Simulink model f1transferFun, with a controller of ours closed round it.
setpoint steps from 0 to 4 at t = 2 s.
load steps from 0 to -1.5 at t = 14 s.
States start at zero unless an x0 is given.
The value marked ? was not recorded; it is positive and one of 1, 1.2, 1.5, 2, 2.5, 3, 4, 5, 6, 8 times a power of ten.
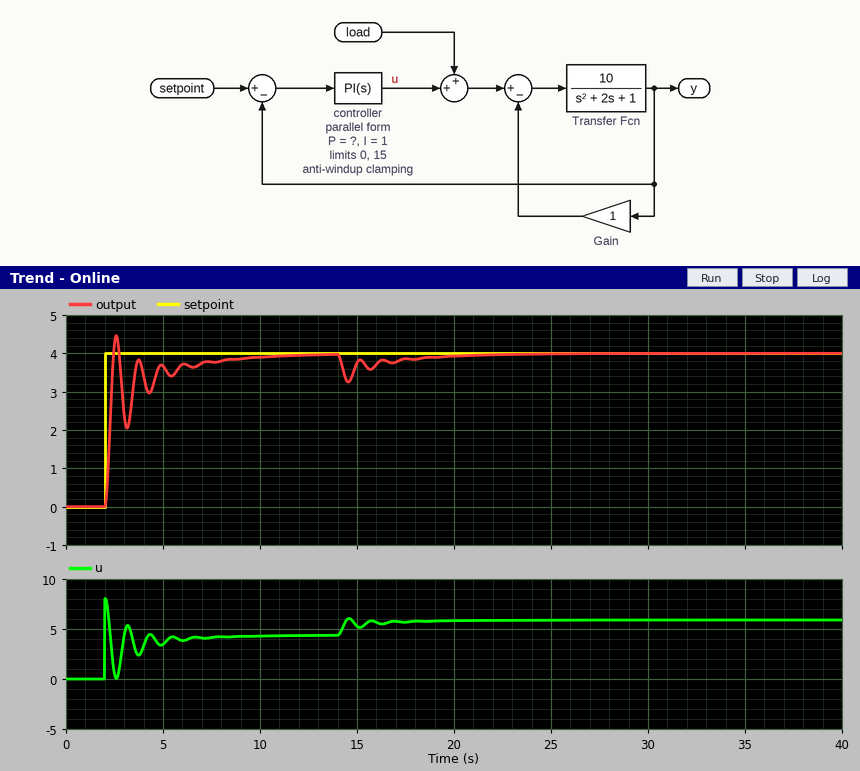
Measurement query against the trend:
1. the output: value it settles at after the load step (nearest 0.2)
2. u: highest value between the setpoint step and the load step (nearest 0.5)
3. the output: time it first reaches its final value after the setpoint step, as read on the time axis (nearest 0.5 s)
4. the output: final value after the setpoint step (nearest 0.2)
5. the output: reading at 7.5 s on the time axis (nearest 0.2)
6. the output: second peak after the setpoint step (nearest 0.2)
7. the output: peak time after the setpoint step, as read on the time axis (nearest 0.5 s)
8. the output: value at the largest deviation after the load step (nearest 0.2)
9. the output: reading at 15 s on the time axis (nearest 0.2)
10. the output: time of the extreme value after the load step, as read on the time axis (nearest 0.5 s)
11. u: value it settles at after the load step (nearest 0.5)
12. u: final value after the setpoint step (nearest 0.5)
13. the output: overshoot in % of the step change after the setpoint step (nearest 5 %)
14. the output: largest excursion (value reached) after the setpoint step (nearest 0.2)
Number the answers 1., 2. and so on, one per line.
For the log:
1. 4.0
2. 8.0
3. 2.5 s
4. 4.0
5. 3.8
6. 3.8
7. 2.5 s
8. 3.2
9. 3.8
10. 14.5 s
11. 6.0
12. 4.5
13. 10 %
14. 4.4
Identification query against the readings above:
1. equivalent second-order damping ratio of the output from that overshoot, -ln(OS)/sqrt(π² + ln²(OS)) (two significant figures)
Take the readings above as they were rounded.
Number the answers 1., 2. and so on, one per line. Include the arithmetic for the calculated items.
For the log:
1. ln(0.1) = -2.303; 2.303 / sqrt(9.870 + 5.302) = 0.59
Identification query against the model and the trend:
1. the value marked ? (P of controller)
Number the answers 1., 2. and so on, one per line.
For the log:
1. 2
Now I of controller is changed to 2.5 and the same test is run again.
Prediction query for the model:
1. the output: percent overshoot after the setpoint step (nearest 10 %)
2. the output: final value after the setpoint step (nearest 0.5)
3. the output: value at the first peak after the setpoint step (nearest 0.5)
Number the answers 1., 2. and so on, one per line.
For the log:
1. 30 %
2. 4.0
3. 5.0
